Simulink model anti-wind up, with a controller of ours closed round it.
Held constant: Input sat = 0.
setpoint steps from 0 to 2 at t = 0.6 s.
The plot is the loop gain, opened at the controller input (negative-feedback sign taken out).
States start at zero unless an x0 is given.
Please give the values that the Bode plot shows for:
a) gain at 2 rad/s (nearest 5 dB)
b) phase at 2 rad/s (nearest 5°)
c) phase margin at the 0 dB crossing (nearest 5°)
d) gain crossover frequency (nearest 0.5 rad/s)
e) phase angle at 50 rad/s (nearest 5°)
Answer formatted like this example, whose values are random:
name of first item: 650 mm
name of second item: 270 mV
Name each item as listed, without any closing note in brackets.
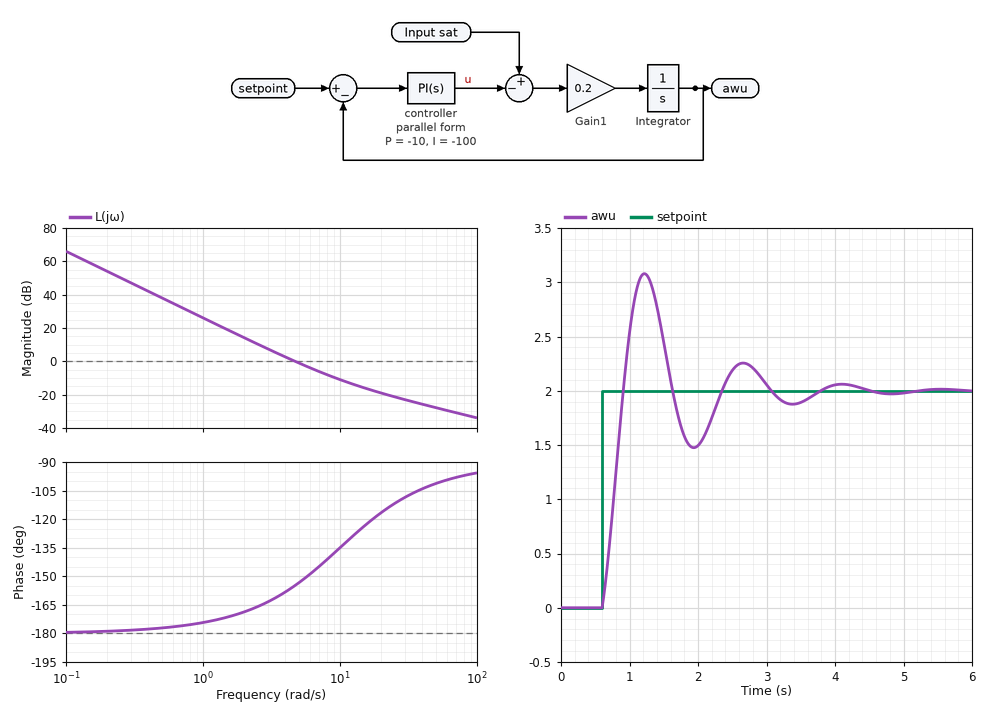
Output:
gain at 2 rad/s: 15 dB
phase at 2 rad/s: -170°
phase margin at the 0 dB crossing: 25°
gain crossover frequency: 4.5 rad/s
phase angle at 50 rad/s: -100°
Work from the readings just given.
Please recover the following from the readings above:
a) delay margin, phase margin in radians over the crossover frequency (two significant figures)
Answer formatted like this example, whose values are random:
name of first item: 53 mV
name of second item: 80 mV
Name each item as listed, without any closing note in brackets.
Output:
delay margin, phase margin in radians over the crossover frequency: 0.097 s
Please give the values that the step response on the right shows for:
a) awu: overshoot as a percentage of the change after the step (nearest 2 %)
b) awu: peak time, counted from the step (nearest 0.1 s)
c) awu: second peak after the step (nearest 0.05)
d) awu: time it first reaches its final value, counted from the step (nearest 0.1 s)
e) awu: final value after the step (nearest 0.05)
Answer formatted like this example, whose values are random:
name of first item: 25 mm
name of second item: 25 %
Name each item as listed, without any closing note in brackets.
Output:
awu: overshoot as a percentage of the change after the step: 54 %
awu: peak time, counted from the step: 0.6 s
awu: second peak after the step: 2.25
awu: time it first reaches its final value, counted from the step: 0.3 s
awu: final value after the step: 2.00
